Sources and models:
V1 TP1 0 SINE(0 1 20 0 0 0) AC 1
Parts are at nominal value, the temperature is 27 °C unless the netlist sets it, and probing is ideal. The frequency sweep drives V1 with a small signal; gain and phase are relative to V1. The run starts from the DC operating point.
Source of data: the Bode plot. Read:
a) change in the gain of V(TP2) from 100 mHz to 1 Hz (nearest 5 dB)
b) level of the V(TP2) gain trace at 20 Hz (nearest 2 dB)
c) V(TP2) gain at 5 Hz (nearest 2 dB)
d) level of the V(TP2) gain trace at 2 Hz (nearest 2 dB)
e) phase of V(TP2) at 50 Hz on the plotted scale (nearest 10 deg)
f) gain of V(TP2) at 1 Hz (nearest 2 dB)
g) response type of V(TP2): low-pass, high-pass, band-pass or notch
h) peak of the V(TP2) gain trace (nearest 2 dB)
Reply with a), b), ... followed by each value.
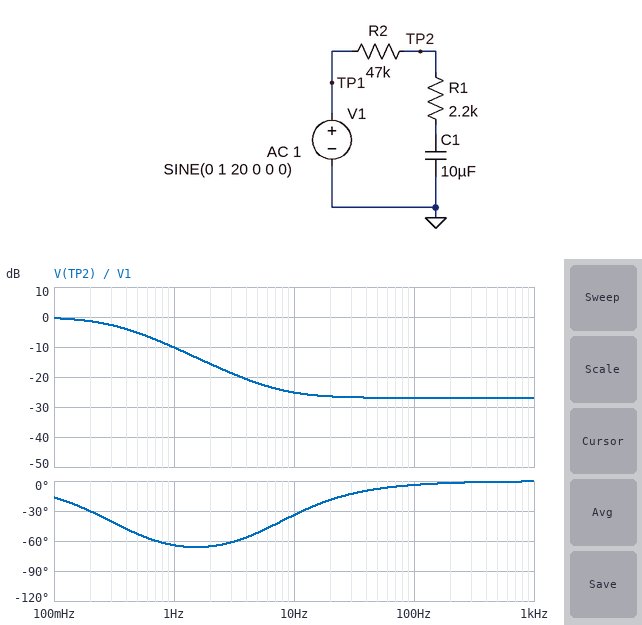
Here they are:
a) -10 dB
b) -26 dB
c) -22 dB
d) -16 dB
e) -10 deg
f) -10 dB
g) low-pass
h) 0 dB
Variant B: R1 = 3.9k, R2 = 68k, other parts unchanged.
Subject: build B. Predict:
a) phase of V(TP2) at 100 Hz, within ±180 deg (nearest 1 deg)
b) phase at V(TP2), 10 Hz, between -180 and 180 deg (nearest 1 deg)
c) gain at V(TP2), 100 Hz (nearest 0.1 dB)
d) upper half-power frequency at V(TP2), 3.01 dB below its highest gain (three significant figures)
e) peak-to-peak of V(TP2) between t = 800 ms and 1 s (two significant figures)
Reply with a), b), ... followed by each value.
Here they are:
a) -2 deg
b) -21 deg
c) -25.3 dB
d) 222 mHz
e) 110 mV
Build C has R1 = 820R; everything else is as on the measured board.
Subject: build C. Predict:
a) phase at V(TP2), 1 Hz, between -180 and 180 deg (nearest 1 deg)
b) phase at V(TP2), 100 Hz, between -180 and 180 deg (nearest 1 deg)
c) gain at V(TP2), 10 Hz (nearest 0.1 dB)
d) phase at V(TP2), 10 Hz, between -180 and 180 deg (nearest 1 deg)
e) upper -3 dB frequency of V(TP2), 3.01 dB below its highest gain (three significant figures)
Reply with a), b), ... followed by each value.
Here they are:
a) -69 deg
b) -11 deg
c) -28.5 dB
d) -61 deg
e) 333 mHz
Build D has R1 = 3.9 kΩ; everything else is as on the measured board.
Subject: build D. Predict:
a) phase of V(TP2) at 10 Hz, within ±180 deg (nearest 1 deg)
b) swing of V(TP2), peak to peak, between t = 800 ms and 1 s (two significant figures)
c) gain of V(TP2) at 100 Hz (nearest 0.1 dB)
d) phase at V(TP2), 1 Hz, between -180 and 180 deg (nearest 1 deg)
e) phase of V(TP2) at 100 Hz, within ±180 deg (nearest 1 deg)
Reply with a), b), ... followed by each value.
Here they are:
a) -20 deg
b) 160 mV
c) -22.3 dB
d) -59 deg
e) -2 deg
